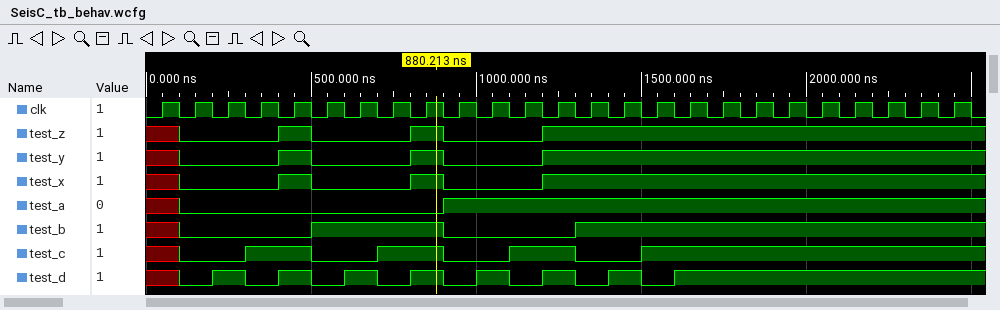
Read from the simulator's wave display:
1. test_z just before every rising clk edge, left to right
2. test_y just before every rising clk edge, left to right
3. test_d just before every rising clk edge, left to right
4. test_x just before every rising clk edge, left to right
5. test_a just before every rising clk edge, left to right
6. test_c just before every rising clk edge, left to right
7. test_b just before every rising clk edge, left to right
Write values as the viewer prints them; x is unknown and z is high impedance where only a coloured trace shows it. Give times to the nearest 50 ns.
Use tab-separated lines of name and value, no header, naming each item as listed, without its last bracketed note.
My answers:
test_z just before every rising clk edge, left to right	x 0 0 0 1 0 0 0 1 0 0 0 1 1 1 1 1 1 1 1 1 1 1 1 1
test_y just before every rising clk edge, left to right	x 0 0 0 1 0 0 0 1 0 0 0 1 1 1 1 1 1 1 1 1 1 1 1 1
test_d just before every rising clk edge, left to right	x 0 1 0 1 0 1 0 1 0 1 0 1 0 1 0 1 1 1 1 1 1 1 1 1
test_x just before every rising clk edge, left to right	x 0 0 0 1 0 0 0 1 0 0 0 1 1 1 1 1 1 1 1 1 1 1 1 1
test_a just before every rising clk edge, left to right	x 0 0 0 0 0 0 0 0 1 1 1 1 1 1 1 1 1 1 1 1 1 1 1 1
test_c just before every rising clk edge, left to right	x 0 0 1 1 0 0 1 1 0 0 1 1 0 0 1 1 1 1 1 1 1 1 1 1
test_b just before every rising clk edge, left to right	x 0 0 0 0 1 1 1 1 0 0 0 0 1 1 1 1 1 1 1 1 1 1 1 1
